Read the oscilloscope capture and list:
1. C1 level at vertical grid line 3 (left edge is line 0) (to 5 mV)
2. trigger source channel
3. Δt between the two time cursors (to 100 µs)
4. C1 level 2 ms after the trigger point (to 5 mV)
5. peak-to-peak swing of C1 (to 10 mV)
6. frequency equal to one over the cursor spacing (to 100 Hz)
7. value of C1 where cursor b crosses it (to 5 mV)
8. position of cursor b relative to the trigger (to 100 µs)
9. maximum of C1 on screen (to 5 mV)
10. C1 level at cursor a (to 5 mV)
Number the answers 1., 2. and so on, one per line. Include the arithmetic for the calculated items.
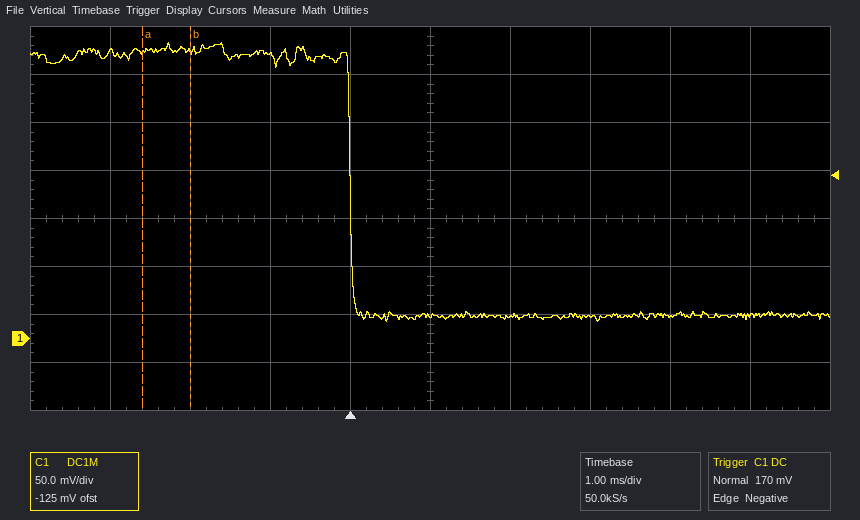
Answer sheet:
1. 295 mV
2. C1
3. 600 µs
4. 25 mV
5. 290 mV
6. 1 / 600 µs ≈ 1.7 kHz
7. 300 mV
8. -2.0 ms
9. 310 mV
10. 300 mV
